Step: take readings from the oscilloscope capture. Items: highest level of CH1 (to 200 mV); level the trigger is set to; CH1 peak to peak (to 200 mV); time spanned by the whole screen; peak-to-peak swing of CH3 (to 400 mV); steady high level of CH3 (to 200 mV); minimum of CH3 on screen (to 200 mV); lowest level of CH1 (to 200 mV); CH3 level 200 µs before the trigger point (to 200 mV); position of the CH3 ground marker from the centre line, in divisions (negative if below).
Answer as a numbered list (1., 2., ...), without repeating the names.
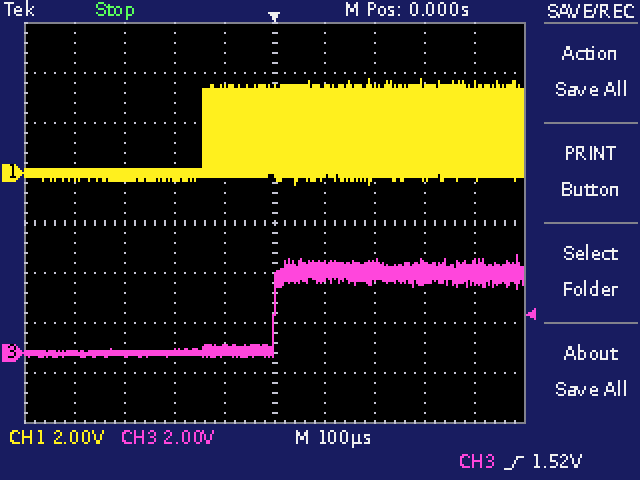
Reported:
1. 3.8 V
2. 1.52 V
3. 4.2 V
4. 1 ms
5. 4.0 V
6. 3.2 V
7. -200 mV
8. -400 mV
9. 0.0 V
10. -2.6 div
